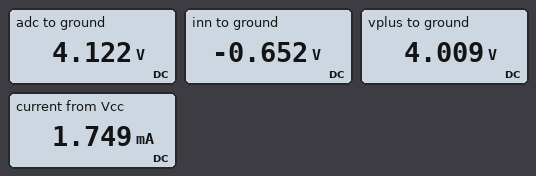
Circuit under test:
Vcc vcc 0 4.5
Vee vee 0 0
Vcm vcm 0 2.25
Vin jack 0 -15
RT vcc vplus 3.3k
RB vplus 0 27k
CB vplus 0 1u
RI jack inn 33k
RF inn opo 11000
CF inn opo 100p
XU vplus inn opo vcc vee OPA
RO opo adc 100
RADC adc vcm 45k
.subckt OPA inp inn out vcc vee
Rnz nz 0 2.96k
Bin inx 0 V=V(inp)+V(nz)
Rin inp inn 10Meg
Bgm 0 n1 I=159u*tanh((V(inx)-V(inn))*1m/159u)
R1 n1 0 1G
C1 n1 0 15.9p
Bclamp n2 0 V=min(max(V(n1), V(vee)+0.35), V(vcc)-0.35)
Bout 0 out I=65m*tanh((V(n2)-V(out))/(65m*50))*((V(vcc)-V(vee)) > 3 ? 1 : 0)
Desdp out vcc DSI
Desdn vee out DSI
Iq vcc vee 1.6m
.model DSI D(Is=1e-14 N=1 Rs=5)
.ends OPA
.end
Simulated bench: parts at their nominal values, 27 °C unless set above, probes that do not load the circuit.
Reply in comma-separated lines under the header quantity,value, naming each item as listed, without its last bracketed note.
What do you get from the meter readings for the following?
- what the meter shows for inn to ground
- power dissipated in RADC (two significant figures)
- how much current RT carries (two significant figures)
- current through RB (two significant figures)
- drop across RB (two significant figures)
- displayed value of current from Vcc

quantity,value
what the meter shows for inn to ground,-0.652 V
power dissipated in RADC,78 µW
how much current RT carries,150 µA
current through RB,150 µA
drop across RB,4.0 V
displayed value of current from Vcc,1.749 mA
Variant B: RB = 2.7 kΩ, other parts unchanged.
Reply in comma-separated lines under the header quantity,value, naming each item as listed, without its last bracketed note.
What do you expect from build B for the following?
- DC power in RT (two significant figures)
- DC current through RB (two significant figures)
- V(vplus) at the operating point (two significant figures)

quantity,value
DC power in RT,1.9 mW
DC current through RB,750 µA
V(vplus) at the operating point,2.0 V
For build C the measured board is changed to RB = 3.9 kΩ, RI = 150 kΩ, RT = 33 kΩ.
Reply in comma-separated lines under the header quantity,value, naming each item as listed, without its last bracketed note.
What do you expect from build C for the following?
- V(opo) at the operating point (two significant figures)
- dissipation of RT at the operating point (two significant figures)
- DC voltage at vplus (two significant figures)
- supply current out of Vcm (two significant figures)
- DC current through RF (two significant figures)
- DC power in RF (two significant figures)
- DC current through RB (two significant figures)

quantity,value
V(opo) at the operating point,1.6 V
dissipation of RT at the operating point,490 µW
DC voltage at vplus,480 mV
supply current out of Vcm,14 µA
DC current through RF,100 µA
DC power in RF,120 µW
DC current through RB,120 µA
